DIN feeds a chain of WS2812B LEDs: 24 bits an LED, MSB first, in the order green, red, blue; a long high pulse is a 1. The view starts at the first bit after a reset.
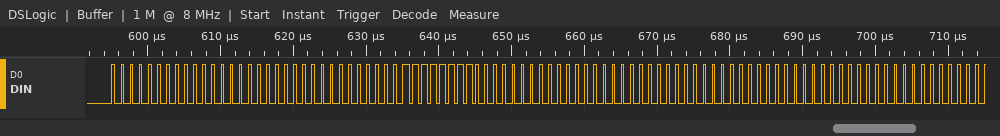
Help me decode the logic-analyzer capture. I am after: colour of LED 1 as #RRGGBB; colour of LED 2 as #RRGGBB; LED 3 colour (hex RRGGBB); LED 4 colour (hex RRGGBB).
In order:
#000000
#FF0000
#000000
#000000
